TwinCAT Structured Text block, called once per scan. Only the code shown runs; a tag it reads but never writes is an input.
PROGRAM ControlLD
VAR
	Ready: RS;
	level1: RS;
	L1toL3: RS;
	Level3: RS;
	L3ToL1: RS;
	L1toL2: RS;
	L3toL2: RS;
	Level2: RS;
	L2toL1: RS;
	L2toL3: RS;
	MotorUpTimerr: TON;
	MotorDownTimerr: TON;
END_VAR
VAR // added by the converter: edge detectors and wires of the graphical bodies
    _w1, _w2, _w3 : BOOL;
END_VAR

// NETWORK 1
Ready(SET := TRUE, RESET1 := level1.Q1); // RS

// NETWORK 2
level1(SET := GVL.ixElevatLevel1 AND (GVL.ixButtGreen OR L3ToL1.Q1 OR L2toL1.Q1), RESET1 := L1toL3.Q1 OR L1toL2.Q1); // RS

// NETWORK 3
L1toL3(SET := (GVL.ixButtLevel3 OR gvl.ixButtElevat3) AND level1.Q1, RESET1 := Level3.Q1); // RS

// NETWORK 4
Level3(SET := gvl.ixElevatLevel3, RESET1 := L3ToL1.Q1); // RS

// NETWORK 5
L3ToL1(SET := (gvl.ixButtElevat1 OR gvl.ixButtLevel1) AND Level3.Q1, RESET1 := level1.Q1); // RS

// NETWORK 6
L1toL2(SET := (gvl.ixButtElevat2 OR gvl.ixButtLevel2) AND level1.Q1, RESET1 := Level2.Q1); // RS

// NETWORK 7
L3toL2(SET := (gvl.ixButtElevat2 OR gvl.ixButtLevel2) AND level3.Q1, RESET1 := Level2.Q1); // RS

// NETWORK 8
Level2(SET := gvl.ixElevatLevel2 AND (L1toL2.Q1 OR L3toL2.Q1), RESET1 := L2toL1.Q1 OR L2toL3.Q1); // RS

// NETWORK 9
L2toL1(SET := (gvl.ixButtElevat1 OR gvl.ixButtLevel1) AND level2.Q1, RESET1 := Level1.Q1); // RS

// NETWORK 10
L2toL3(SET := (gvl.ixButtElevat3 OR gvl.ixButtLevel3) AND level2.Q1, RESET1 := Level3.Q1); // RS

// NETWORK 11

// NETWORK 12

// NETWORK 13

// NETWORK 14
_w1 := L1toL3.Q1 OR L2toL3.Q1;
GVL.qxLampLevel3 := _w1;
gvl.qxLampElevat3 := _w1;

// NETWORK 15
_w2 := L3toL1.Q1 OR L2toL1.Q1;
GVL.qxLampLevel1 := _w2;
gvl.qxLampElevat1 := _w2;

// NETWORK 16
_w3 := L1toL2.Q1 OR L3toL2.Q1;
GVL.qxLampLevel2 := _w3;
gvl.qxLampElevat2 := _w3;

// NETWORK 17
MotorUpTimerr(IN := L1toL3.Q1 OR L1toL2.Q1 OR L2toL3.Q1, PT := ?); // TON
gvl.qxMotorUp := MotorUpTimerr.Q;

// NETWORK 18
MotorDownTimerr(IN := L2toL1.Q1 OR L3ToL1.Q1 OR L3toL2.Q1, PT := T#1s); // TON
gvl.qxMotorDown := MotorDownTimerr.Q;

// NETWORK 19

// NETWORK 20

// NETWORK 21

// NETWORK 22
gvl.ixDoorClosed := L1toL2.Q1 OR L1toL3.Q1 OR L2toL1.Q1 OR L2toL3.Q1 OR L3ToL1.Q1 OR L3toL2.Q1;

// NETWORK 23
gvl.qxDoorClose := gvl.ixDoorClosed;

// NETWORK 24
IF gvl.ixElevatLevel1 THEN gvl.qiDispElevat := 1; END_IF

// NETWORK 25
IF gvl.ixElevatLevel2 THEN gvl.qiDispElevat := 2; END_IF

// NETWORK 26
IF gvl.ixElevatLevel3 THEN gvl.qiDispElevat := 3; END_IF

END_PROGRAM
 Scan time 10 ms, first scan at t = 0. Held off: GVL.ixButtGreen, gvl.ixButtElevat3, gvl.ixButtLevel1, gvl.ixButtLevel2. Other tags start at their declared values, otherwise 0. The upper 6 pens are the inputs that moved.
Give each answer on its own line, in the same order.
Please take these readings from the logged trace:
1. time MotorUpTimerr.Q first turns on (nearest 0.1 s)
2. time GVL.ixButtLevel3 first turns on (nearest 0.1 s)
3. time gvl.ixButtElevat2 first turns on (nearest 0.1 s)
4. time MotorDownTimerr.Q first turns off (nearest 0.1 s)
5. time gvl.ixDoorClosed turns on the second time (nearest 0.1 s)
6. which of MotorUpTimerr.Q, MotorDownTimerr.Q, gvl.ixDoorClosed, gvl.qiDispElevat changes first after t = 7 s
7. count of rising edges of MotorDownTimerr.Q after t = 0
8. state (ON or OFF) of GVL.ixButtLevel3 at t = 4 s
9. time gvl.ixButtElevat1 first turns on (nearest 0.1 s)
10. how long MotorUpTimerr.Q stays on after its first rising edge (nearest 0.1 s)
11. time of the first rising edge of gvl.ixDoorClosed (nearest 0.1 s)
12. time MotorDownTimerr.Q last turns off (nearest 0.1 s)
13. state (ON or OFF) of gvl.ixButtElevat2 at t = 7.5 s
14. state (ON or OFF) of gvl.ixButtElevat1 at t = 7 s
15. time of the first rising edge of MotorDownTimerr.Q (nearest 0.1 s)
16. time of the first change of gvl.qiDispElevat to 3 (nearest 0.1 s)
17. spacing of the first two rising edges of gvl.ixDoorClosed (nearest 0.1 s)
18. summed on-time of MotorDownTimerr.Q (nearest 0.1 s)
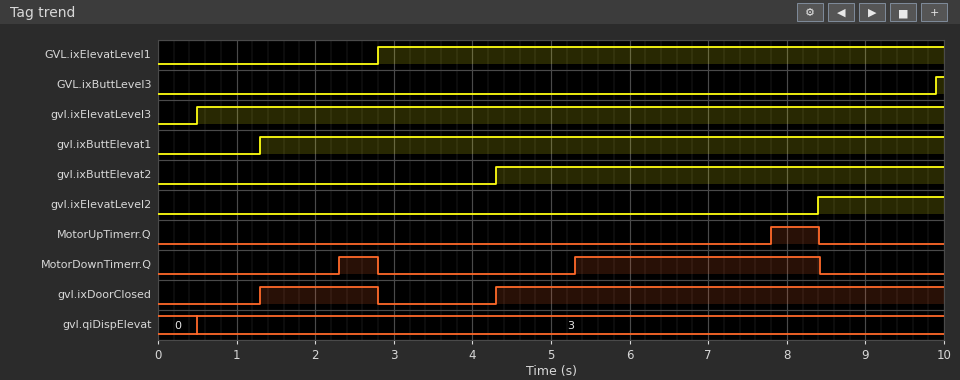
7.8 s
9.9 s
4.3 s
2.8 s
4.3 s
MotorUpTimerr.Q
2
OFF
1.3 s
0.6 s
1.3 s
8.4 s
ON
ON
2.3 s
0.5 s
3.0 s
3.6 s
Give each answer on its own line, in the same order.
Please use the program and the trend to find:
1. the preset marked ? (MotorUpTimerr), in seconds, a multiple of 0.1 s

3.5 s
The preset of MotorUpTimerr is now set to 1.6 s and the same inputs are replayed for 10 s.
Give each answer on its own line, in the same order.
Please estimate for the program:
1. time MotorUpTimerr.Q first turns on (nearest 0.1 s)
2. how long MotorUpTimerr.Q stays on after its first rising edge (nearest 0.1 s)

5.9 s
2.5 s
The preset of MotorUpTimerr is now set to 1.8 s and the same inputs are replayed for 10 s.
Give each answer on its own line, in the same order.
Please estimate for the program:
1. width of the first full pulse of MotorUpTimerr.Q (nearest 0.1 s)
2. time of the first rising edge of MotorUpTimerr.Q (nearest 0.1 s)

2.3 s
6.1 s
